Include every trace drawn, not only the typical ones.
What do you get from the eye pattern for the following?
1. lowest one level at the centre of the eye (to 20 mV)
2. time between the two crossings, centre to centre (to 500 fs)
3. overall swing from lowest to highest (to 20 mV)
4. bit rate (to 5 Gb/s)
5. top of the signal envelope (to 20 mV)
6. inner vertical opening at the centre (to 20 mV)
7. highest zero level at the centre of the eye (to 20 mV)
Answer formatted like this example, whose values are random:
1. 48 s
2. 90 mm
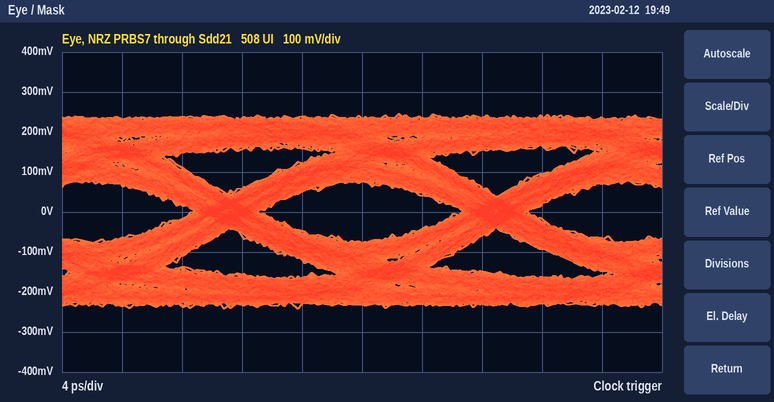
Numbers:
1. 80 mV
2. 18.0 ps
3. 480 mV
4. 55 Gb/s
5. 240 mV
6. 160 mV
7. -80 mV
